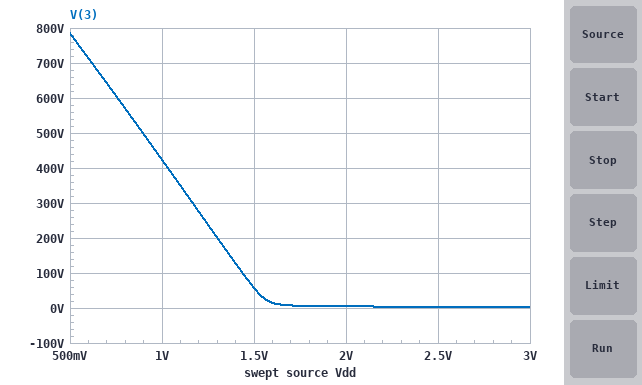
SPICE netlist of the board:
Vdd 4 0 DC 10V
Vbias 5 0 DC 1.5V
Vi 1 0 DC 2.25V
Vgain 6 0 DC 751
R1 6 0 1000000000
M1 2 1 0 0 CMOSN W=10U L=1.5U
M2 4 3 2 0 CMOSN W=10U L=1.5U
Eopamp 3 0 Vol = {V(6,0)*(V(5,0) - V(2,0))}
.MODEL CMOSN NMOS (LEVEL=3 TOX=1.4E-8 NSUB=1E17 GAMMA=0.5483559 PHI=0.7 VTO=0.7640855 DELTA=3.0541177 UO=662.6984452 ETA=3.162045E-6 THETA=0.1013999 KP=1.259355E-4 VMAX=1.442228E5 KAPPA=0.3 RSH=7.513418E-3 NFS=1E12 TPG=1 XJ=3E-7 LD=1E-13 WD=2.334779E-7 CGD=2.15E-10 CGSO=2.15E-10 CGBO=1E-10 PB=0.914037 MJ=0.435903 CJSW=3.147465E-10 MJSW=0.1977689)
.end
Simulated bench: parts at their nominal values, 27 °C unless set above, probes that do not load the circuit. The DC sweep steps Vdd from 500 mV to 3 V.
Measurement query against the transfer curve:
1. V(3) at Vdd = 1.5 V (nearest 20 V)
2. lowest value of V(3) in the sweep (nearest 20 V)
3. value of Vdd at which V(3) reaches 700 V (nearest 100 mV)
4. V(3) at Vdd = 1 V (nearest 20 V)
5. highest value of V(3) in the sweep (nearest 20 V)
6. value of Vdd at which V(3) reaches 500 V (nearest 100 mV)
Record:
60 V
0 V
600 mV
420 V
780 V
900 mV
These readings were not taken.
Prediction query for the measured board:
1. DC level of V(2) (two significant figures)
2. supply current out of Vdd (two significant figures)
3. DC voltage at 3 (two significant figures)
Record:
1.5 V
510 µA
4.0 V
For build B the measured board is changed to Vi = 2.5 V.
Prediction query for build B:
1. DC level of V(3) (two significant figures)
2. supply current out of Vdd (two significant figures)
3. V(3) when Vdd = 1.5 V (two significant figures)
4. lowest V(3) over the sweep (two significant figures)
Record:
4.2 V
660 µA
72 V
4.3 V
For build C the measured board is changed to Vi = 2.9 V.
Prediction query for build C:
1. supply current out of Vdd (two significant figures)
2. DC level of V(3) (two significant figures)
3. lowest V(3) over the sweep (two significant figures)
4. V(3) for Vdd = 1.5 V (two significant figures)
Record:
910 µA
4.5 V
4.7 V
95 V
